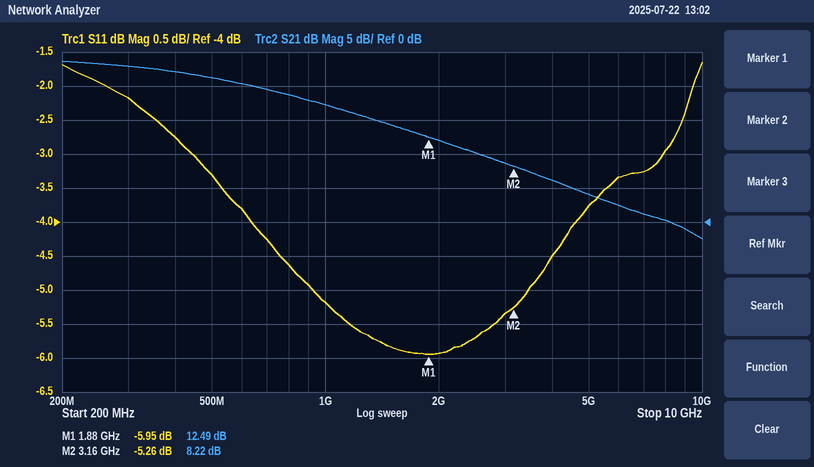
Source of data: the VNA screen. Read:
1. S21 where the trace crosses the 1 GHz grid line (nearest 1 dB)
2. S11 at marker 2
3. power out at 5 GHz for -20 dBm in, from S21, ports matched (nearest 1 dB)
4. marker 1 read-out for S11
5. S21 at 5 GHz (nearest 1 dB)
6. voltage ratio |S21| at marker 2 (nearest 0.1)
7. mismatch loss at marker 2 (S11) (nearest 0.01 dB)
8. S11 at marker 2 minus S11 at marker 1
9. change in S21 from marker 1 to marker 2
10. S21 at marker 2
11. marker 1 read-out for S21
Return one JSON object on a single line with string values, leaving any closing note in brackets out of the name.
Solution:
{"S21 where the trace crosses the 1 GHz grid line": "17 dB", "S11 at marker 2": "-5.26 dB", "power out at 5 GHz for -20 dBm in, from S21, ports matched": "-16 dBm", "marker 1 read-out for S11": "-5.95 dB", "S21 at 5 GHz": "4 dB", "voltage ratio |S21| at marker 2": "2.6", "mismatch loss at marker 2 (S11)": "1.54 dB", "S11 at marker 2 minus S11 at marker 1": "0.69 dB", "change in S21 from marker 1 to marker 2": "-4.27 dB", "S21 at marker 2": "8.22 dB", "marker 1 read-out for S21": "12.49 dB"}
